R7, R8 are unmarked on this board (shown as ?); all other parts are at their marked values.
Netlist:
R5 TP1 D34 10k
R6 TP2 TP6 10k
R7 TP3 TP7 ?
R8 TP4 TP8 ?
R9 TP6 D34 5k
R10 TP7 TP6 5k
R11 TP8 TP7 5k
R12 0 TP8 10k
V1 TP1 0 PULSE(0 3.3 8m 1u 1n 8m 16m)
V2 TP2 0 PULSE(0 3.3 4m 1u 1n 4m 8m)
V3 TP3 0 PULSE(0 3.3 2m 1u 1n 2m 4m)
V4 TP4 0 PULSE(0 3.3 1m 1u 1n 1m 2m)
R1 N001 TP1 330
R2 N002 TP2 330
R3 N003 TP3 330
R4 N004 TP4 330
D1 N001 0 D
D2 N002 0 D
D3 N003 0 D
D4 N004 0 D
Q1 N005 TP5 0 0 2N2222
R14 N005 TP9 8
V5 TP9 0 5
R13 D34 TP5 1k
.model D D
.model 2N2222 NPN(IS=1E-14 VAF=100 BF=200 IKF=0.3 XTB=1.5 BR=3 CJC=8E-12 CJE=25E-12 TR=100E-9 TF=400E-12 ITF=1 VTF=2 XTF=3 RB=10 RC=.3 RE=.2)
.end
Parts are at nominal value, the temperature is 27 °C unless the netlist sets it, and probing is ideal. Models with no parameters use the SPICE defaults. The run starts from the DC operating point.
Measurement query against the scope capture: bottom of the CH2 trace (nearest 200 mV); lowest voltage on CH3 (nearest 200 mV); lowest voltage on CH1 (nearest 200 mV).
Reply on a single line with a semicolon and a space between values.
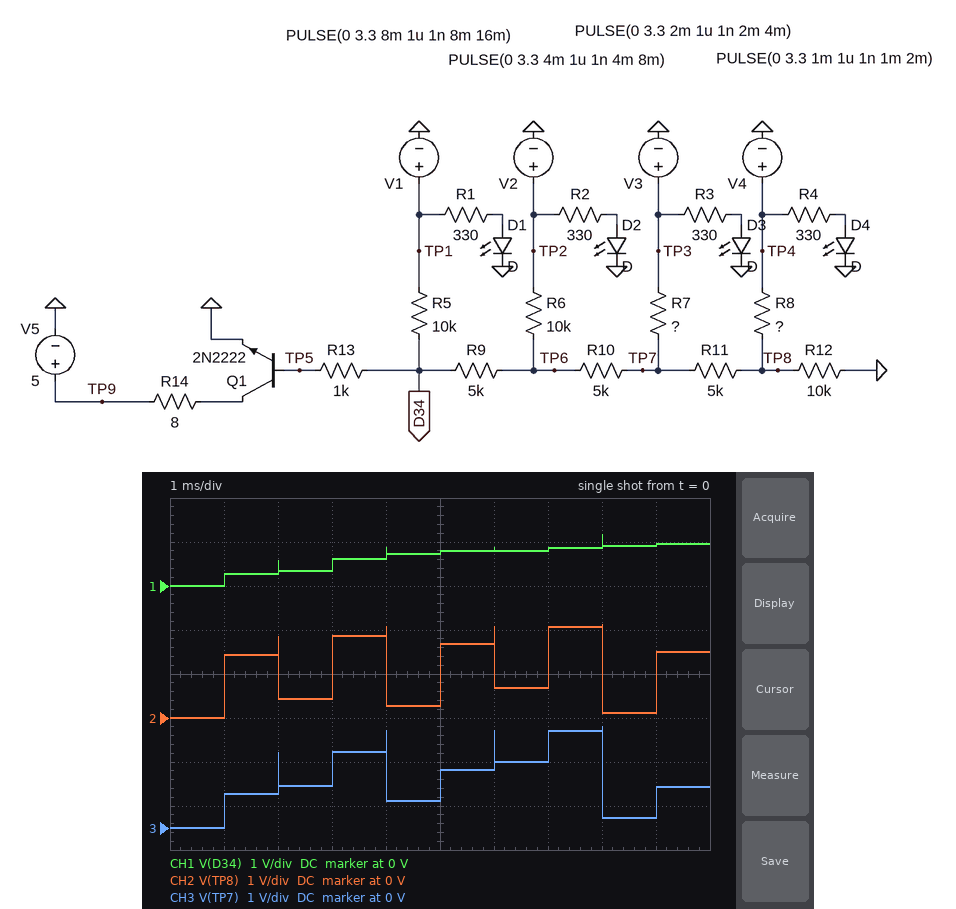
0 V; 0 V; 0 V
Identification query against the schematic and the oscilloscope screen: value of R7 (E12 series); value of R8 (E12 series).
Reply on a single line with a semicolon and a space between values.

12 kΩ; 6.8 kΩ
